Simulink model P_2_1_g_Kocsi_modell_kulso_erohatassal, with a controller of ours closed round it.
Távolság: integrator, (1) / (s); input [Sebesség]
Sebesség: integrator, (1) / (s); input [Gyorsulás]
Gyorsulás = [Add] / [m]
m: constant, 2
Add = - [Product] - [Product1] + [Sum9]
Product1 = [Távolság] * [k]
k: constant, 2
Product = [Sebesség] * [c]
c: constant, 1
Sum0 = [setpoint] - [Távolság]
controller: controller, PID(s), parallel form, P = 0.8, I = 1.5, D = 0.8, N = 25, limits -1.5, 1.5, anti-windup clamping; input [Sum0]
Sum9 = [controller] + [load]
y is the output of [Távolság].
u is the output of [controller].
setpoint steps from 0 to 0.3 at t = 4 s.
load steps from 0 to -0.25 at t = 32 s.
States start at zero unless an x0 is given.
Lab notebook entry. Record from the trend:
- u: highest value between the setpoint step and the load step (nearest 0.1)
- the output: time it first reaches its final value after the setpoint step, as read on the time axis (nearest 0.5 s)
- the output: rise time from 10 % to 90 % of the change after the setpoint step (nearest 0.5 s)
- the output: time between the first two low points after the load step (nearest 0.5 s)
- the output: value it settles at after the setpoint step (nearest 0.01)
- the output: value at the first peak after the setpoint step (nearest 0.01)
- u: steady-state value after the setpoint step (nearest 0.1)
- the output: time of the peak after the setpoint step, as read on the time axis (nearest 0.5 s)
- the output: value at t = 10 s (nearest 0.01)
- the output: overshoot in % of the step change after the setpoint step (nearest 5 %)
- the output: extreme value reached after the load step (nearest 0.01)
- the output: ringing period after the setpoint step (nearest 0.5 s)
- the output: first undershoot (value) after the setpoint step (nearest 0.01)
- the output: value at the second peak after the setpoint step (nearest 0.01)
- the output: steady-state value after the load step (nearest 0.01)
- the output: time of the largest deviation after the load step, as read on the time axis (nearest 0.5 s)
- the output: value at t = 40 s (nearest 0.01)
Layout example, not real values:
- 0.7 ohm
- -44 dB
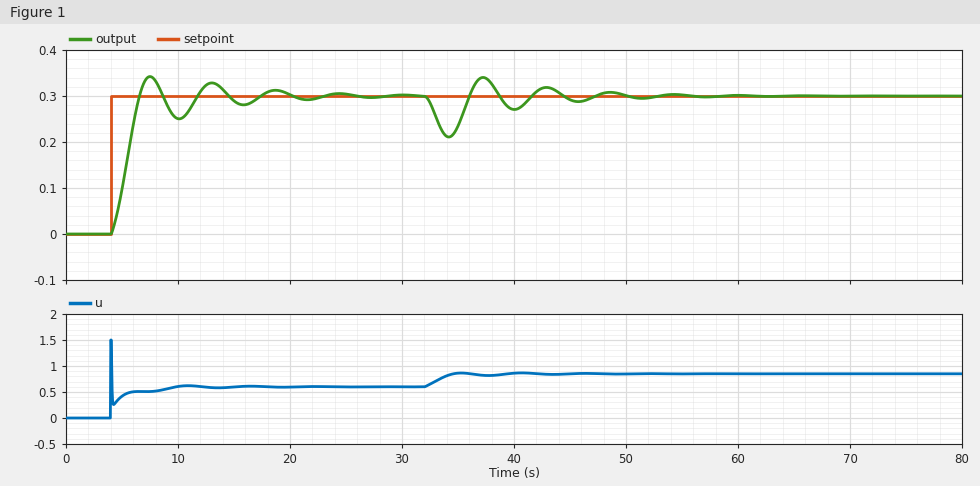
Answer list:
- 1.5
- 6.5 s
- 2.0 s
- 6.0 s
- 0.30
- 0.34
- 0.6
- 7.5 s
- 0.25
- 15 %
- 0.21
- 5.5 s
- 0.25
- 0.33
- 0.30
- 34.0 s
- 0.27
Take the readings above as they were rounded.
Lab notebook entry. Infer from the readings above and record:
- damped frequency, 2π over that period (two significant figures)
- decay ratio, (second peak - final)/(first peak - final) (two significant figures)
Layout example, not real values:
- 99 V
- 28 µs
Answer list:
- 1.1 rad/s
- 0.75
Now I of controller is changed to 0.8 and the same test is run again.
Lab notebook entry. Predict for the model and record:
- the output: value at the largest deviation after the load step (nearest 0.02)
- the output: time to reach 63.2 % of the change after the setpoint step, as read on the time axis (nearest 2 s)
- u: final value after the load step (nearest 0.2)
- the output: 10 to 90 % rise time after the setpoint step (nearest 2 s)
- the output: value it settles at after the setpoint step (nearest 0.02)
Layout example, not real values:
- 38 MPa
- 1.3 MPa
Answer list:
- 0.20
- 6 s
- 0.8
- 6 s
- 0.30
